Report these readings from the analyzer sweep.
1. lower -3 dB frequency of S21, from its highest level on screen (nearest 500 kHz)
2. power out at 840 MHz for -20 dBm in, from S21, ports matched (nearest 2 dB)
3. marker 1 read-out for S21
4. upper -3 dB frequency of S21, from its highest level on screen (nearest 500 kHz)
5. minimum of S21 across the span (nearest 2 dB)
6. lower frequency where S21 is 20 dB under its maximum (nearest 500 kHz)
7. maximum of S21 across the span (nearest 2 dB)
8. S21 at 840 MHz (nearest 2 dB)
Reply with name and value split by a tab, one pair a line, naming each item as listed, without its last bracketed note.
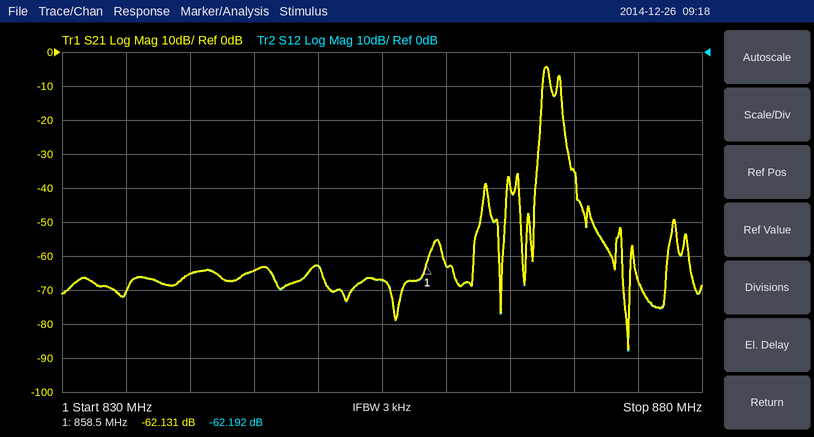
lower -3 dB frequency of S21, from its highest level on screen	867.5 MHz
power out at 840 MHz for -20 dBm in, from S21, ports matched	-86 dBm
marker 1 read-out for S21	-62.131 dB
upper -3 dB frequency of S21, from its highest level on screen	868.0 MHz
minimum of S21 across the span	-88 dB
lower frequency where S21 is 20 dB under its maximum	867.5 MHz
maximum of S21 across the span	-4 dB
S21 at 840 MHz	-66 dB
